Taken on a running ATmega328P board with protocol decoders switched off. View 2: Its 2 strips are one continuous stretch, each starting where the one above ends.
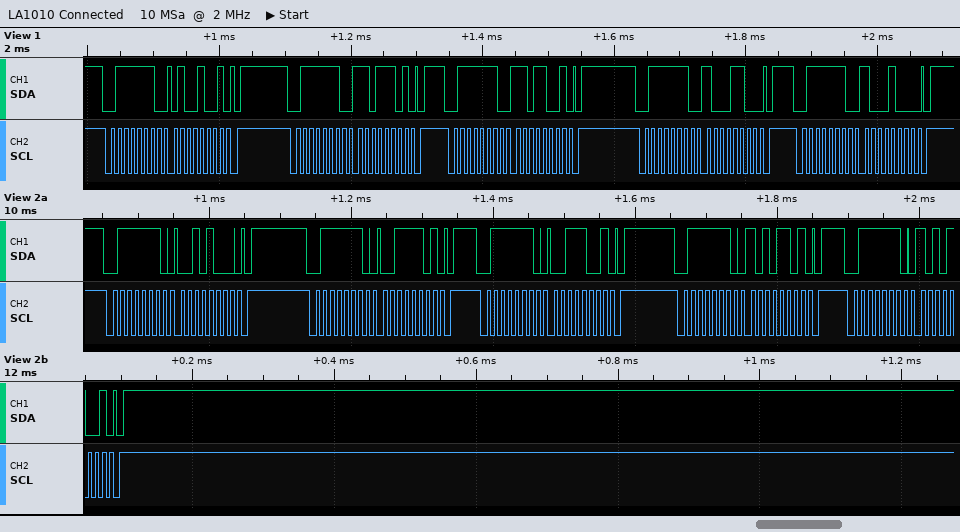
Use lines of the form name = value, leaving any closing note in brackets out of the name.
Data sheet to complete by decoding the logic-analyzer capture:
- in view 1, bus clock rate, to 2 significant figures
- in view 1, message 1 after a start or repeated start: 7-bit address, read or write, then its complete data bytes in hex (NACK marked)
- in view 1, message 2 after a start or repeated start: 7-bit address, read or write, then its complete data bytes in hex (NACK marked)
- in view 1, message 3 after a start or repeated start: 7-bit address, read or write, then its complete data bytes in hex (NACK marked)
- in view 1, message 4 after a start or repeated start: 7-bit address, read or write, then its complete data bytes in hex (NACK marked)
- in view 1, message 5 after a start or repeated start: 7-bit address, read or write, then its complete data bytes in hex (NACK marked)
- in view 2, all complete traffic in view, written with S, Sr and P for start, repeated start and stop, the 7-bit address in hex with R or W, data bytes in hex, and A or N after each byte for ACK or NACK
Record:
in view 1, bus clock rate, to 2 significant figures = 100 kHz
in view 1, message 1 after a start or repeated start: 7-bit address, read or write, then its complete data bytes in hex = 0x3F write: 49
in view 1, message 2 after a start or repeated start: 7-bit address, read or write, then its complete data bytes in hex = 0x3F write: DD
in view 1, message 3 after a start or repeated start: 7-bit address, read or write, then its complete data bytes in hex = 0x3F write: D9
in view 1, message 4 after a start or repeated start: 7-bit address, read or write, then its complete data bytes in hex = 0x3F write: 8C
in view 1, message 5 after a start or repeated start: 7-bit address, read or write, then its complete data bytes in hex = 0x3F write: 88
in view 2, all complete traffic in view, written with S, Sr and P for start, repeated start and stop, the 7-bit address in hex with R or W, data bytes in hex, and A or N after each byte for ACK or NACK = S 3FW A 28 A P S 3FW A 3D A P S 3FW A 39 A P S 3FW A AD A P S 3FW A A9 A P
